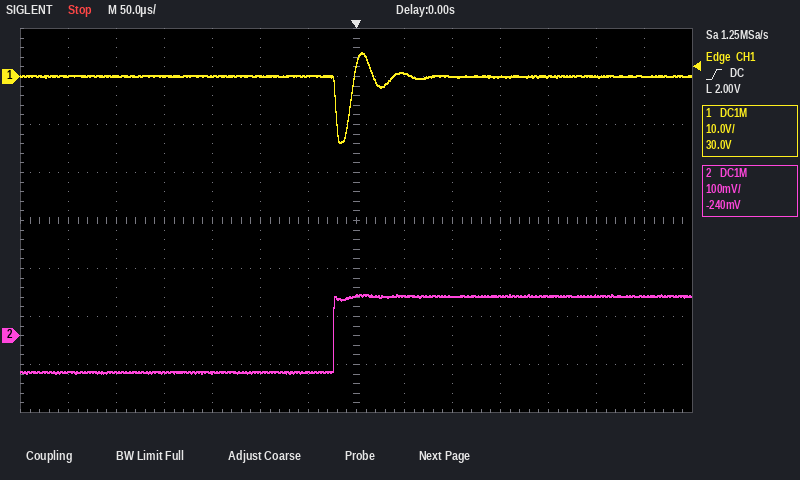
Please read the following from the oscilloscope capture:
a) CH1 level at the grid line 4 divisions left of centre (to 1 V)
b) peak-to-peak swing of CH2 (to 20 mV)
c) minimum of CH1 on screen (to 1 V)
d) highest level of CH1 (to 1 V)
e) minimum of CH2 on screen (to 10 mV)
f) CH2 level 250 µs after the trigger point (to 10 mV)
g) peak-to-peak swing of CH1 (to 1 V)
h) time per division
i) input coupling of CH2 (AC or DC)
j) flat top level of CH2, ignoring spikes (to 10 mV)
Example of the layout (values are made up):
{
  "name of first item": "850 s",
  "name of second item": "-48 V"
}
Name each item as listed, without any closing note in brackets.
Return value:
{
  "CH1 level at the grid line 4 divisions left of centre": "0 V",
  "peak-to-peak swing of CH2": "160 mV",
  "minimum of CH1 on screen": "-14 V",
  "highest level of CH1": "5 V",
  "minimum of CH2 on screen": "-80 mV",
  "CH2 level 250 µs after the trigger point": "80 mV",
  "peak-to-peak swing of CH1": "19 V",
  "time per division": "50 µs",
  "input coupling of CH2": "DC",
  "flat top level of CH2, ignoring spikes": "80 mV"
}
